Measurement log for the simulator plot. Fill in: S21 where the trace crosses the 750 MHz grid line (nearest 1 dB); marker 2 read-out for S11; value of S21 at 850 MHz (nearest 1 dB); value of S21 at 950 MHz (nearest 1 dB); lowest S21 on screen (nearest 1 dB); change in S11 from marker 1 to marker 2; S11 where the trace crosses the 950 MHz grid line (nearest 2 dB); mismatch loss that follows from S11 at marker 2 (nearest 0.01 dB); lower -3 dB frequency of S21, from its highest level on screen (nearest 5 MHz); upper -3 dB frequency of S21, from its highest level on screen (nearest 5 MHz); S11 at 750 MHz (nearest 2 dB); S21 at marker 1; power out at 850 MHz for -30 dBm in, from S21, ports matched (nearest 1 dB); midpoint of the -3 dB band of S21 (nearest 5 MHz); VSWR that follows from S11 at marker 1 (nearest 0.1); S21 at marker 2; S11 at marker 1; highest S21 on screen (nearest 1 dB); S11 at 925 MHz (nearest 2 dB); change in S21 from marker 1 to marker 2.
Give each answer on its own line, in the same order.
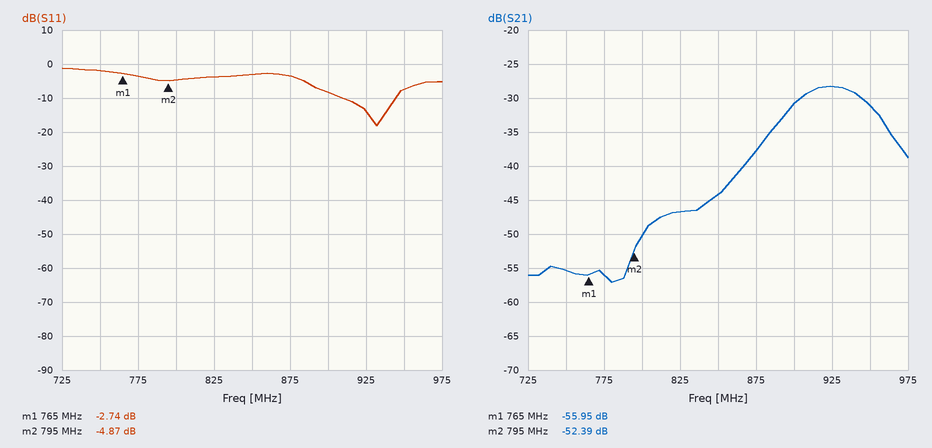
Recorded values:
-55 dB
-4.87 dB
-44 dB
-31 dB
-57 dB
-2.13 dB
-8 dB
1.71 dB
900 MHz
950 MHz
-2 dB
-55.95 dB
-74 dBm
925 MHz
6.4
-52.39 dB
-2.74 dB
-28 dB
-14 dB
3.56 dB
